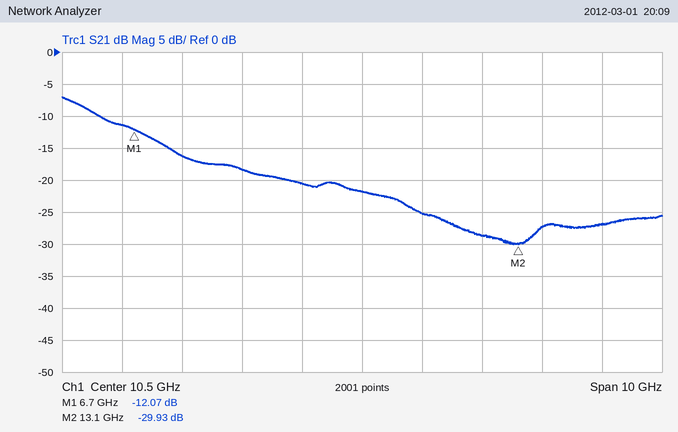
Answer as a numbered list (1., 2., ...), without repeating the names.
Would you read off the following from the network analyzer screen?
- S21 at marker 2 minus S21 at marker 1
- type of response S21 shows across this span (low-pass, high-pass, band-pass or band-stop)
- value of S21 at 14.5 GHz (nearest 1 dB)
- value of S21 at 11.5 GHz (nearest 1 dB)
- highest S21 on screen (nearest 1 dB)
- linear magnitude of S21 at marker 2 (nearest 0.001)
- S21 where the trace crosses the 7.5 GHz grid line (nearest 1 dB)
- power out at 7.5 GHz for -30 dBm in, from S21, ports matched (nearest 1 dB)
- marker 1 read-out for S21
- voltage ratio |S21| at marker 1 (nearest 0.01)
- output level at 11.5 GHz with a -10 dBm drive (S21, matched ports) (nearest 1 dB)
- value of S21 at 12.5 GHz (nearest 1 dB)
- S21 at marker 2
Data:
1. -17.86 dB
2. low-pass
3. -27 dB
4. -25 dB
5. -7 dB
6. 0.032
7. -16 dB
8. -46 dBm
9. -12.07 dB
10. 0.25
11. -35 dBm
12. -29 dB
13. -29.93 dB
